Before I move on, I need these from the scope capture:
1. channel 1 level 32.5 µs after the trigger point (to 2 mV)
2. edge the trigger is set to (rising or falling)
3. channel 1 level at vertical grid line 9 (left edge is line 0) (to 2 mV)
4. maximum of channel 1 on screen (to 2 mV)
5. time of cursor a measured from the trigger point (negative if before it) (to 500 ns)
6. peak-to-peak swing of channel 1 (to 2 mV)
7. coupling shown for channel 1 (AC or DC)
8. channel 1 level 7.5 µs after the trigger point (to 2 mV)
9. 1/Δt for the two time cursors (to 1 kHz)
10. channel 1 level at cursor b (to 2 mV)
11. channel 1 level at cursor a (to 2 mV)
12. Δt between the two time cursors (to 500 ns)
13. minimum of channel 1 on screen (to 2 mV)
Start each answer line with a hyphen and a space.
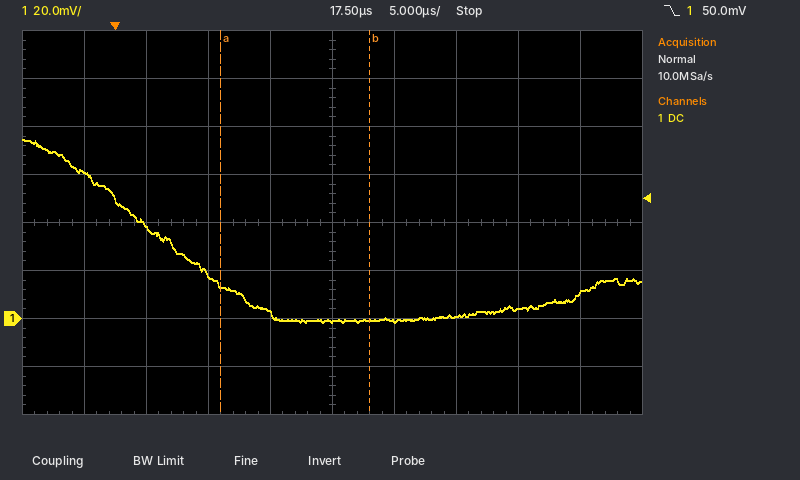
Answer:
- 4 mV
- falling
- 10 mV
- 74 mV
- +8.5 µs
- 76 mV
- DC
- 18 mV
- 83 kHz
- 0 mV
- 14 mV
- 12.0 µs
- -2 mV
